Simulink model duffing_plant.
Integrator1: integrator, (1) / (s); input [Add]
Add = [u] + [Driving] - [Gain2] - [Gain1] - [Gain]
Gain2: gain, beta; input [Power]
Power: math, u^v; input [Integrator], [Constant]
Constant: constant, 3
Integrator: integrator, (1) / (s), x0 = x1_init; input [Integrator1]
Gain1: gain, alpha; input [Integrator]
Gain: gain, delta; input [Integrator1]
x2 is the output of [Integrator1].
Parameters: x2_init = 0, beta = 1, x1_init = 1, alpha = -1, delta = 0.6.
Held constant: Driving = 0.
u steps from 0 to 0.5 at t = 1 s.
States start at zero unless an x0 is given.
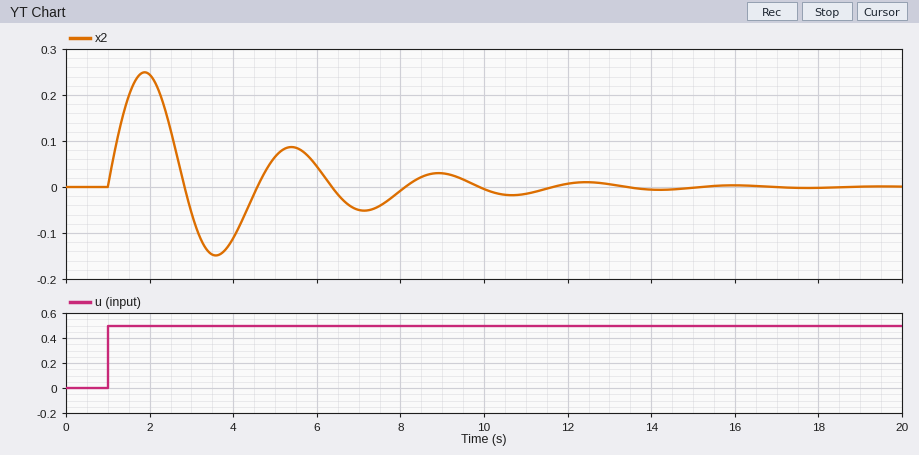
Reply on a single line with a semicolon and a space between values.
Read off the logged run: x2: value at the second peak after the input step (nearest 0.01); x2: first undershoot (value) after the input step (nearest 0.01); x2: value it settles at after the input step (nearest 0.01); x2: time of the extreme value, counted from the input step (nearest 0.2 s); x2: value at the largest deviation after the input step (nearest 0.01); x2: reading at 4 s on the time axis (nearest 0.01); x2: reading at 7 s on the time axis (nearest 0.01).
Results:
0.09; -0.15; 0.00; 0.8 s; 0.25; -0.11; -0.05
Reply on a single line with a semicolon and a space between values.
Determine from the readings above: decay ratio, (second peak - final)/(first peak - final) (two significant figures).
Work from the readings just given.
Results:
0.36
